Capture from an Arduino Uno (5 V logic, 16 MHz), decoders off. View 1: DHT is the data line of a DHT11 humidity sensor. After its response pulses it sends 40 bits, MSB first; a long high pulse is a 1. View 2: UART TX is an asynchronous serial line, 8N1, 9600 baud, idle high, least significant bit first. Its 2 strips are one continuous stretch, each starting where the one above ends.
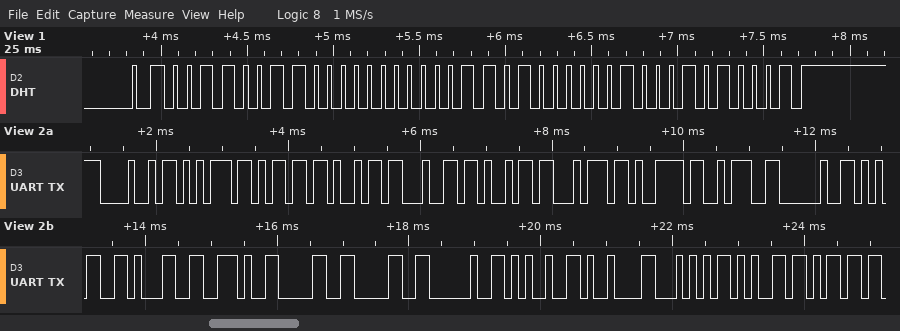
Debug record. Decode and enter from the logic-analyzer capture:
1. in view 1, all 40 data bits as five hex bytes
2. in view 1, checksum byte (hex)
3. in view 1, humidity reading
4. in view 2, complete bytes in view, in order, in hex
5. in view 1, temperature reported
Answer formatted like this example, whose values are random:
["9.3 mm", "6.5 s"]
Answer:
["33 00 1A 04 51", "0x51", "51 %", "48 75 6D 69 64 69 74 79 3A 20 35 31 2E 30 30 20 25 09 54 65 6D", "26.4 °C"]
